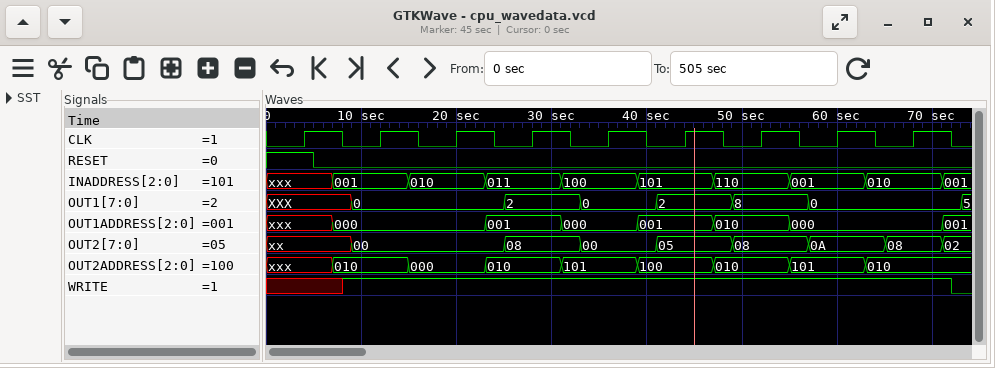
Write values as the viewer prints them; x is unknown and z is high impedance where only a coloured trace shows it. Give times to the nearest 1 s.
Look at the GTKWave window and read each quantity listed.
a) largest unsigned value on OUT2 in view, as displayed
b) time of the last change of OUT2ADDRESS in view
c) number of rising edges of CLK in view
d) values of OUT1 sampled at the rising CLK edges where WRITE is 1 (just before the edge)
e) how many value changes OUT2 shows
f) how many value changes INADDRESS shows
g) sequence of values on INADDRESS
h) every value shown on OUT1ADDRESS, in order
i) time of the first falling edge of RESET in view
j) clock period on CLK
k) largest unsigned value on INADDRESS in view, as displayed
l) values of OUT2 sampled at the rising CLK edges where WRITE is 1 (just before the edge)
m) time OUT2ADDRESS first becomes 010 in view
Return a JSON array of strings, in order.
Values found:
["0A", "63 s", "9", "0, 0, 2, 0, 2, 8, 0, 0", "8", "9", "xxx, 001, 010, 011, 100, 101, 110, 001, 010, 001", "xxx, 000, 001, 000, 001, 010, 000, 001", "5 s", "8 s", "110", "00, 00, 08, 00, 05, 08, 0A, 08", "7 s"]
